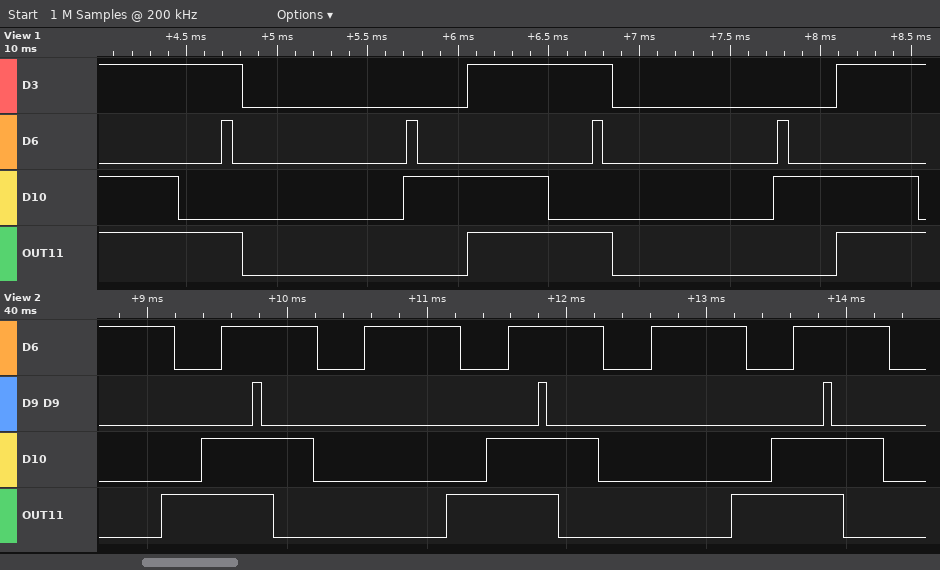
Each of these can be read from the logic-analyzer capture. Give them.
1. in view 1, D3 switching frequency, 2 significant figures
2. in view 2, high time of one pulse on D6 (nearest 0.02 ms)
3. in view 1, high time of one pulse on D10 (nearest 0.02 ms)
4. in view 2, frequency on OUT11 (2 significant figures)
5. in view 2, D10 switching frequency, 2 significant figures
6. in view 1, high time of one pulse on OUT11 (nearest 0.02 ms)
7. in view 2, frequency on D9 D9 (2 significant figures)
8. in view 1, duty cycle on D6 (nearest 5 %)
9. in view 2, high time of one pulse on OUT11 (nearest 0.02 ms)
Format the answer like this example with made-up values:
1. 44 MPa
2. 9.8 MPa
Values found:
1. 490 Hz
2. 0.68 ms
3. 0.80 ms
4. 490 Hz
5. 490 Hz
6. 0.80 ms
7. 490 Hz
8. 5 %
9. 0.80 ms
